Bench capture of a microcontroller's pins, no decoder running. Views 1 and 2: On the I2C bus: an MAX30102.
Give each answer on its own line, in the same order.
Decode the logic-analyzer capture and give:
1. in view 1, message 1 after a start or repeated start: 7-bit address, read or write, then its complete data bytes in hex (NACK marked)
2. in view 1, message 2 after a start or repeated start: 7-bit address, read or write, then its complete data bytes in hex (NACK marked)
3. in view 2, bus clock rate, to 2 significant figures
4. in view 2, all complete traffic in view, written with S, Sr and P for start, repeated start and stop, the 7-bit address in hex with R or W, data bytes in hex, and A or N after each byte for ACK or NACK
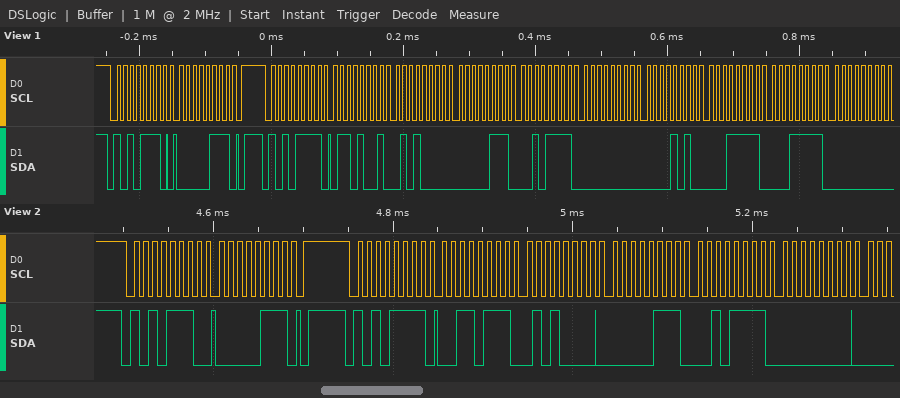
0x57 write: 07
0x57 read: 69 50 07 2F 00 0A 1F 1F 00
100 kHz
S 57W A 07 A P S 57R A 37 A 50 A 07 A 2F A 00 A
